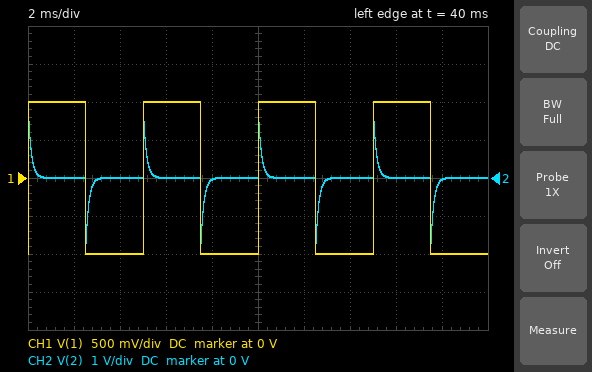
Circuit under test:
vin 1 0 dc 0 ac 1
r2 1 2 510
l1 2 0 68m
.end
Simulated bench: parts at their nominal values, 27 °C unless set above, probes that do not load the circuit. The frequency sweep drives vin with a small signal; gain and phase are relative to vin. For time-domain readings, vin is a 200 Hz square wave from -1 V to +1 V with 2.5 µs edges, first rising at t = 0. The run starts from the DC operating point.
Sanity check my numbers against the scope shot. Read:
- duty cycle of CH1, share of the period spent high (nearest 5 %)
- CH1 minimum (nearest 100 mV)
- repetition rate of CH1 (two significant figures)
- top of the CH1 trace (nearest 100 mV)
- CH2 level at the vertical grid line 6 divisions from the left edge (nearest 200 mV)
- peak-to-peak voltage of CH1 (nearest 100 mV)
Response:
50 %
-1.0 V
200 Hz
1.0 V
0 V
2.0 V
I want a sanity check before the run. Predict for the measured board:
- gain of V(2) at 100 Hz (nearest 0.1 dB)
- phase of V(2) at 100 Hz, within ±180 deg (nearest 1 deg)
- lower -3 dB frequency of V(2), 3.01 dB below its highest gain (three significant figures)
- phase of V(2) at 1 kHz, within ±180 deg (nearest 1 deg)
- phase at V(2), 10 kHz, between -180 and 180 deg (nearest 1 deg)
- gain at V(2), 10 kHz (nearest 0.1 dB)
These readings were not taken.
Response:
-21.6 dB
85 deg
1.19 kHz
50 deg
7 deg
-0.1 dB
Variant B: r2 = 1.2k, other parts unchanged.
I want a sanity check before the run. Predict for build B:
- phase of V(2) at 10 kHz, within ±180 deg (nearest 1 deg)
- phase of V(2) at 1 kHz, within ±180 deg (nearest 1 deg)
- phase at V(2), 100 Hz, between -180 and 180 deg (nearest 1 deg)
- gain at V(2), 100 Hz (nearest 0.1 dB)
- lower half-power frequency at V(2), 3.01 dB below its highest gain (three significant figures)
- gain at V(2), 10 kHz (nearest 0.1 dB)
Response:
16 deg
70 deg
88 deg
-29.0 dB
2.81 kHz
-0.3 dB
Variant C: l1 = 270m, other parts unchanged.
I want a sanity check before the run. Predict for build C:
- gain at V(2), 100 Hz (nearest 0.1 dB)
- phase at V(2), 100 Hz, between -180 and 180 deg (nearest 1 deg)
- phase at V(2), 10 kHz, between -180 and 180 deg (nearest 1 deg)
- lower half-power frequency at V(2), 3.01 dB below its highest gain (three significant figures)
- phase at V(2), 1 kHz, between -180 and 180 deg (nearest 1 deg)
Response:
-10.0 dB
72 deg
2 deg
301 Hz
17 deg
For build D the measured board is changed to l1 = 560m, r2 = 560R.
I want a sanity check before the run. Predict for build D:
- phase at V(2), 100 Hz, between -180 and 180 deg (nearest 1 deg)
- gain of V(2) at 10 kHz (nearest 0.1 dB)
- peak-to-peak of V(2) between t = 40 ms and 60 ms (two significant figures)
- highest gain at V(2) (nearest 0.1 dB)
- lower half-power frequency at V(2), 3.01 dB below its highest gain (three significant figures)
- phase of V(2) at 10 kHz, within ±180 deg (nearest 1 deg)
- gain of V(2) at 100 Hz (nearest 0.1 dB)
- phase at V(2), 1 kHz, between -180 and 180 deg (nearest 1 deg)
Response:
58 deg
0 dB
3.7 V
0 dB
159 Hz
1 deg
-5.5 dB
9 deg
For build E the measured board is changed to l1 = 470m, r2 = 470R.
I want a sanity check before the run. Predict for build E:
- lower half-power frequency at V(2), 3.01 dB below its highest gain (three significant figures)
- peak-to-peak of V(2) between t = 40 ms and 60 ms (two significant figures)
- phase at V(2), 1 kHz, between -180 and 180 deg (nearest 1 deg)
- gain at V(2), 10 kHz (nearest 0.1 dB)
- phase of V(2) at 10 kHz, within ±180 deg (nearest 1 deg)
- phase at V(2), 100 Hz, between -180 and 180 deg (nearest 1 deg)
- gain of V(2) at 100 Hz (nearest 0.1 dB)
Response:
159 Hz
3.7 V
9 deg
0 dB
1 deg
58 deg
-5.5 dB
